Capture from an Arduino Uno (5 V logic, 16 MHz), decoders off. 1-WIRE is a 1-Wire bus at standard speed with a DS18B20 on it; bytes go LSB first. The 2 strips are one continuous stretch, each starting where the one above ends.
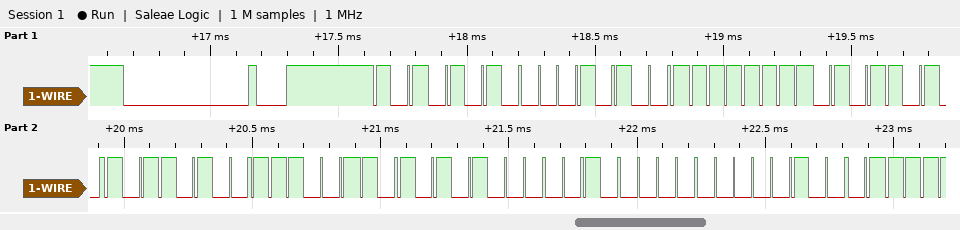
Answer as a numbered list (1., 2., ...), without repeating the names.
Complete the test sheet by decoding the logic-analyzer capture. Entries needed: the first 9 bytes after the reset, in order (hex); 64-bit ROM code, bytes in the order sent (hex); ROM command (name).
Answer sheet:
1. 55 28 FF 5A 2D 67 15 04 20
2. 28 FF 5A 2D 67 15 04 20
3. Match ROM
